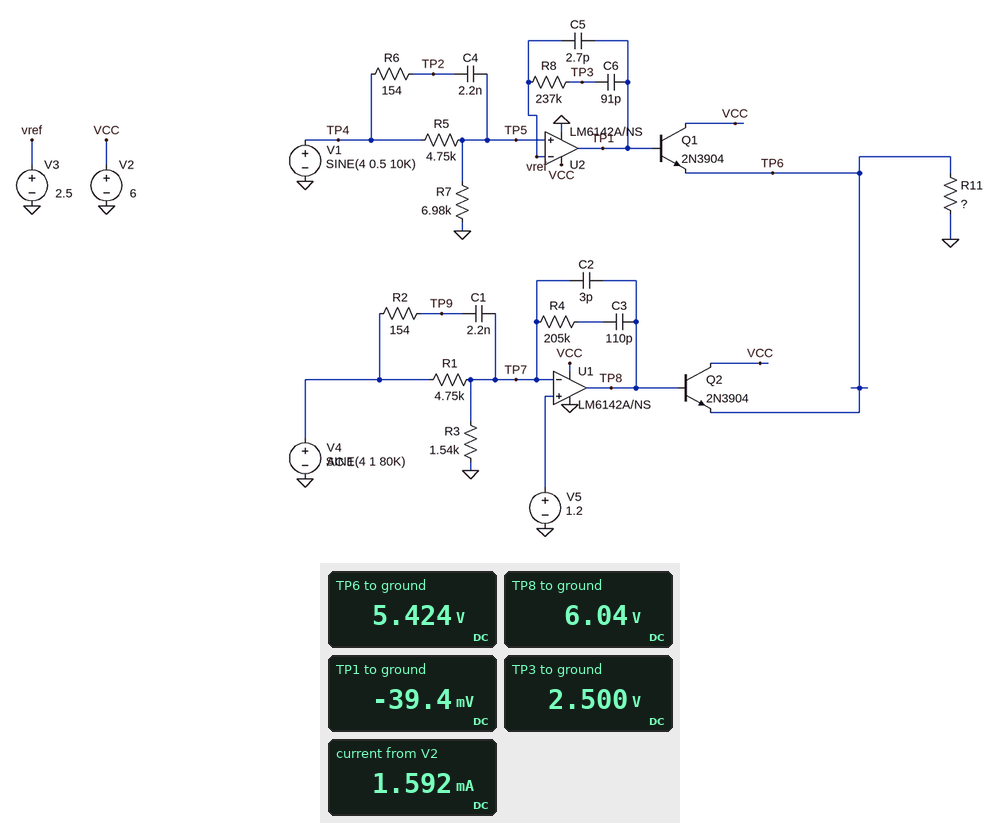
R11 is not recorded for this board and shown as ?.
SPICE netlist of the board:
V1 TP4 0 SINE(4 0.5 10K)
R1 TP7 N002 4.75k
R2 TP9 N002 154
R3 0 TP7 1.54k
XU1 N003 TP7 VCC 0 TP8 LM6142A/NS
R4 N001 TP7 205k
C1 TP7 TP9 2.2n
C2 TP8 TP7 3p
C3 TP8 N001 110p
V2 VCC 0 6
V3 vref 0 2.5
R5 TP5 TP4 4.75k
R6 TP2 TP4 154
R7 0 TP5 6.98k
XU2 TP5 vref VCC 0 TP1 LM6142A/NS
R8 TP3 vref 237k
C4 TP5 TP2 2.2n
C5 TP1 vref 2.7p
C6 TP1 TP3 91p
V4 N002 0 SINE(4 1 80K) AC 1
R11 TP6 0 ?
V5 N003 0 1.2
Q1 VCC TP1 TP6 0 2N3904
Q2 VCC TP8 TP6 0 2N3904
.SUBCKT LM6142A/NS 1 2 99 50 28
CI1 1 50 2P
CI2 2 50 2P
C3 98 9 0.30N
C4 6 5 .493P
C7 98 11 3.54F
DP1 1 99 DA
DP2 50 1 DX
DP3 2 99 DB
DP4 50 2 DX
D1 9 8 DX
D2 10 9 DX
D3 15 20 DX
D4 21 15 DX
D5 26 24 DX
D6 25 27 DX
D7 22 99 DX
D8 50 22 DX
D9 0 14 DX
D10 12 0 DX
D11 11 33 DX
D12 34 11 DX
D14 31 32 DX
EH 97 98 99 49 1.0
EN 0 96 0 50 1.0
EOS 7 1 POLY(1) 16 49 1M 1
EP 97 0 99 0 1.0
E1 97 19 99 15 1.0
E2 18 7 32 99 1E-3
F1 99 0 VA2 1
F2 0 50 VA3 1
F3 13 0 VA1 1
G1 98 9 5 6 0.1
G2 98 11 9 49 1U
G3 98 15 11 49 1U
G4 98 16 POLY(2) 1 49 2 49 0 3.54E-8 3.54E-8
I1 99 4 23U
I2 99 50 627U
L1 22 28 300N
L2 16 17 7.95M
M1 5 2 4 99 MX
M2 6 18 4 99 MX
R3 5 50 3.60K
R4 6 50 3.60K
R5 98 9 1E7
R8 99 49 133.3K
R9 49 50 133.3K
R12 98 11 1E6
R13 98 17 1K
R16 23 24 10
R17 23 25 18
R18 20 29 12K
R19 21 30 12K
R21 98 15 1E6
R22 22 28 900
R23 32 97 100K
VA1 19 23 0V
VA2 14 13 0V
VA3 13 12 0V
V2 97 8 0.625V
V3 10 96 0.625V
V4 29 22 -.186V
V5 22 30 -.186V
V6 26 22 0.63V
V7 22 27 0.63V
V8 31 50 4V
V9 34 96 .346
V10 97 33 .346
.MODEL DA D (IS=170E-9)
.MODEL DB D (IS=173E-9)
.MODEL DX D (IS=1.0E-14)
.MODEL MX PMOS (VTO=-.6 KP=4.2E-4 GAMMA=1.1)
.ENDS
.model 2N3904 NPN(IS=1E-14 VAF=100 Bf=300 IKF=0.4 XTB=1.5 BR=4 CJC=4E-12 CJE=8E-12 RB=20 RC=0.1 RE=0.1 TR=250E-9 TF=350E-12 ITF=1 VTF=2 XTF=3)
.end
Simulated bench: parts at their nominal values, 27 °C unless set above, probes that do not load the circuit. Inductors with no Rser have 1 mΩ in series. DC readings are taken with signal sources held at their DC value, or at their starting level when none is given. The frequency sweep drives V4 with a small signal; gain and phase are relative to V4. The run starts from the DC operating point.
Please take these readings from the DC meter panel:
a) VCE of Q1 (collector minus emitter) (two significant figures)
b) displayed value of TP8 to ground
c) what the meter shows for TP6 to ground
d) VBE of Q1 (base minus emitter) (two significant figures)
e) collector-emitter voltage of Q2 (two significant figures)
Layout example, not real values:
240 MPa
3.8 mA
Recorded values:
580 mV
6.04 V
5.424 V
-5.5 V
580 mV
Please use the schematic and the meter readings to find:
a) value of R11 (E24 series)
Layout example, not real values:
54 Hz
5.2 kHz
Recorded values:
22 kΩ
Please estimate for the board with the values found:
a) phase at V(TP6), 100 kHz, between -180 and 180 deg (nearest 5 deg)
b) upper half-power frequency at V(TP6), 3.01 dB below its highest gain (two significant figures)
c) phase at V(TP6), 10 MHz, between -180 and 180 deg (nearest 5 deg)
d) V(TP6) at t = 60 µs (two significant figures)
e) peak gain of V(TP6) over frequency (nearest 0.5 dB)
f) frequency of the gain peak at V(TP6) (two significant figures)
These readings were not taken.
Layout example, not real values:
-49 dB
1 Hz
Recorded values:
-160 deg
200 MHz
140 deg
5.4 V
-7.5 dB
130 MHz
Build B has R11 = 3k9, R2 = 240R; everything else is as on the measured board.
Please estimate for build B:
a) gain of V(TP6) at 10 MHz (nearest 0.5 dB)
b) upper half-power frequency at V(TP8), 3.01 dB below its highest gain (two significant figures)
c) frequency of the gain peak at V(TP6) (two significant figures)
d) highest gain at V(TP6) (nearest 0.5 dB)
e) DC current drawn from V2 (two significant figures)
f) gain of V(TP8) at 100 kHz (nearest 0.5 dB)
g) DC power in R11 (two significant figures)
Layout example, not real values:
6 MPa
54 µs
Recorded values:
-29.0 dB
180 MHz
97 MHz
-6.5 dB
2.7 mA
-31.5 dB
7.4 mW
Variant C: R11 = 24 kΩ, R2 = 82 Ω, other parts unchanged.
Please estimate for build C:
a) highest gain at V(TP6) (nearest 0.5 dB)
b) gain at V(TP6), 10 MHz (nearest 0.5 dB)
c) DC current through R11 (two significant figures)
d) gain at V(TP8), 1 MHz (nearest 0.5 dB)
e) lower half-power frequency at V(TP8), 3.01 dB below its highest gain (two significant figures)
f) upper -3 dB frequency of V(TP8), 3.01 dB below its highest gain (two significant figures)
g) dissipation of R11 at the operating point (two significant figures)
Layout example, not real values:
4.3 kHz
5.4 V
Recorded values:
-6.5 dB
-28.0 dB
230 µA
-29.5 dB
72 MHz
210 MHz
1.2 mW
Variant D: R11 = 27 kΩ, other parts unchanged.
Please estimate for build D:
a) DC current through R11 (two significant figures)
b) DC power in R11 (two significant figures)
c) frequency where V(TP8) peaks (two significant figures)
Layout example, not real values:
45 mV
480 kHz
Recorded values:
200 µA
1.1 mW
130 MHz
